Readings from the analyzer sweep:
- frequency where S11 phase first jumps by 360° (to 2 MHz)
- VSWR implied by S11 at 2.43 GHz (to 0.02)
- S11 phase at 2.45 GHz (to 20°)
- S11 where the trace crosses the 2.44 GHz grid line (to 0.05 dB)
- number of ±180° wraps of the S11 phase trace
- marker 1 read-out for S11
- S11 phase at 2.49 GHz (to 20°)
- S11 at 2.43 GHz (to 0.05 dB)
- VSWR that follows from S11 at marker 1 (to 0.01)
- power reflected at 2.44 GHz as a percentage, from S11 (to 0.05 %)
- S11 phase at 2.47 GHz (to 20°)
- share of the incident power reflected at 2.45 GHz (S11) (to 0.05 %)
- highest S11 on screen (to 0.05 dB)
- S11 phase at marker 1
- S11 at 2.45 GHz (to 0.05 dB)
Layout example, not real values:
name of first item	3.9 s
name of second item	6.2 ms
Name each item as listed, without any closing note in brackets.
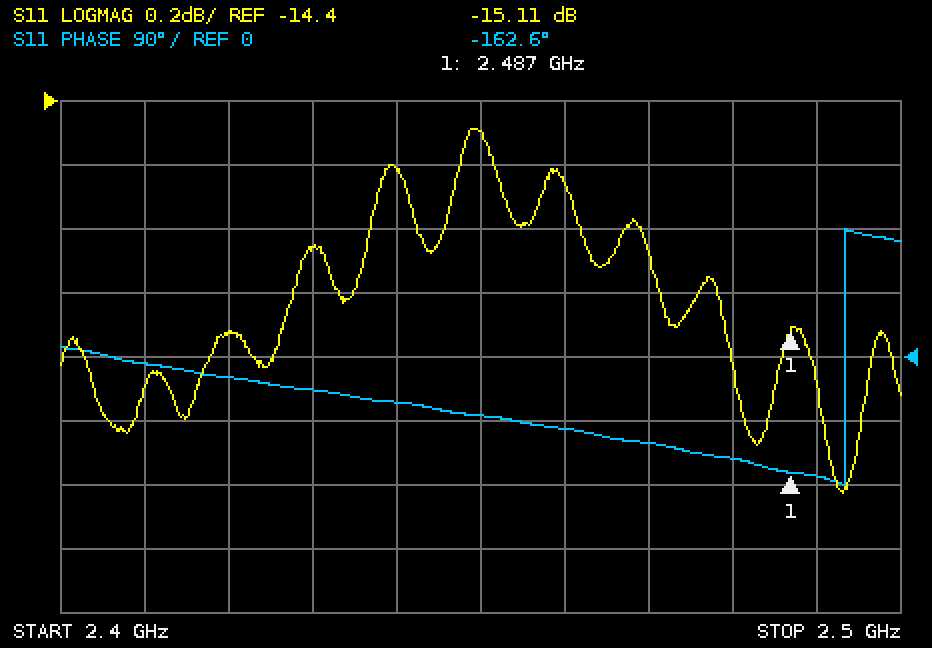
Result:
frequency where S11 phase first jumps by 360°	2.494 GHz
VSWR implied by S11 at 2.43 GHz	1.44
S11 phase at 2.45 GHz	-80°
S11 where the trace crosses the 2.44 GHz grid line	-14.60 dB
number of ±180° wraps of the S11 phase trace	1
marker 1 read-out for S11	-15.11 dB
S11 phase at 2.49 GHz	-160°
S11 at 2.43 GHz	-14.85 dB
VSWR that follows from S11 at marker 1	1.43
power reflected at 2.44 GHz as a percentage, from S11	3.45 %
S11 phase at 2.47 GHz	-120°
share of the incident power reflected at 2.45 GHz (S11)	3.55 %
highest S11 on screen	-14.50 dB
S11 phase at marker 1	-162.6°
S11 at 2.45 GHz	-14.50 dB
